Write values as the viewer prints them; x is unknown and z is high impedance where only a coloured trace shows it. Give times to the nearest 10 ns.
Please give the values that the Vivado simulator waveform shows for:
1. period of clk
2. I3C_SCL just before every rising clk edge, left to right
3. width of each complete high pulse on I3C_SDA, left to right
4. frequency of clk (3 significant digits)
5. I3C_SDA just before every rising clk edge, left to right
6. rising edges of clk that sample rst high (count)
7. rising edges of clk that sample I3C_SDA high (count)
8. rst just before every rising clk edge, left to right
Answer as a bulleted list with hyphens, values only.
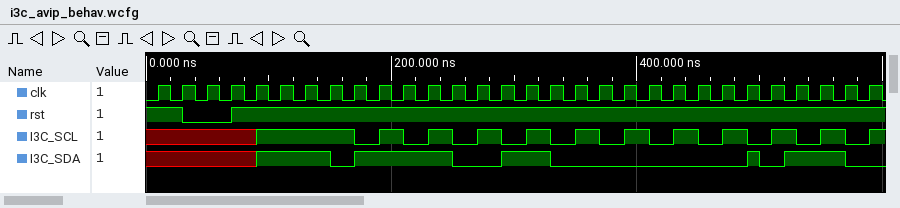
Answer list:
- 20 ns
- x x x x x 1 1 1 1 0 1 0 1 0 1 0 1 0 1 0 1 0 1 0 1 0 1 0 1 0
- 80 ns, 40 ns, 10 ns, 50 ns
- 50.0 MHz
- x x x x x 1 1 1 0 1 1 1 1 0 0 1 1 0 0 0 0 0 0 0 0 0 1 1 1 0
- 28
- 12
- 1 1 0 0 1 1 1 1 1 1 1 1 1 1 1 1 1 1 1 1 1 1 1 1 1 1 1 1 1 1
